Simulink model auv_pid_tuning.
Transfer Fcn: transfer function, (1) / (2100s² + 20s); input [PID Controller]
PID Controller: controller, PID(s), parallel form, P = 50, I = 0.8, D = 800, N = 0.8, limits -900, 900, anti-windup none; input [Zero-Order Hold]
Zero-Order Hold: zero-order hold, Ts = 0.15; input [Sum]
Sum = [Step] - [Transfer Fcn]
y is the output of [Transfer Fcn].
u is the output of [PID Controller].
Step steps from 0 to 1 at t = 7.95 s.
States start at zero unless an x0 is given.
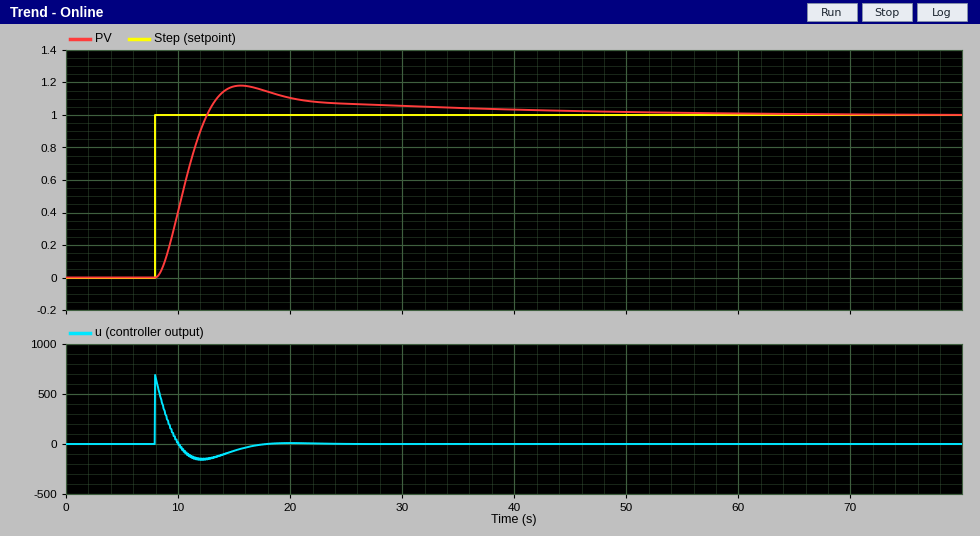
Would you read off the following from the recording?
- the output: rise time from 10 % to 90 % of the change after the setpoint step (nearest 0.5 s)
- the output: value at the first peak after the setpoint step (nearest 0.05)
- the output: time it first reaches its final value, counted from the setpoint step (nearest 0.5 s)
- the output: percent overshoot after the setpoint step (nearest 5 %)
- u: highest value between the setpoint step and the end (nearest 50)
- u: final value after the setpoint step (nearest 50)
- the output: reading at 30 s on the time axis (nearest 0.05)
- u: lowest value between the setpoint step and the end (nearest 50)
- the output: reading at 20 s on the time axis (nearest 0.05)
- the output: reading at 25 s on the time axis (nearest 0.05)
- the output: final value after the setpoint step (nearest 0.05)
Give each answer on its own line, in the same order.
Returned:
3.0 s
1.20
4.5 s
20 %
700
0
1.05
-150
1.10
1.05
1.00
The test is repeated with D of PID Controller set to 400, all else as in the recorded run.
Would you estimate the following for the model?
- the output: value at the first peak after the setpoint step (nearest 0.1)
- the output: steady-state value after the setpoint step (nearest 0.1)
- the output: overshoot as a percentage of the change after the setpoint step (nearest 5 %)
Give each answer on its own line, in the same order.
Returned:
1.3
1.0
30 %
